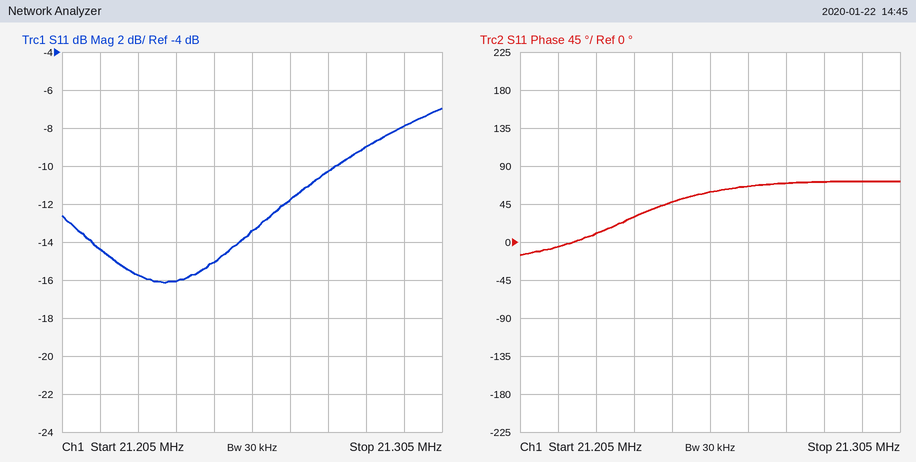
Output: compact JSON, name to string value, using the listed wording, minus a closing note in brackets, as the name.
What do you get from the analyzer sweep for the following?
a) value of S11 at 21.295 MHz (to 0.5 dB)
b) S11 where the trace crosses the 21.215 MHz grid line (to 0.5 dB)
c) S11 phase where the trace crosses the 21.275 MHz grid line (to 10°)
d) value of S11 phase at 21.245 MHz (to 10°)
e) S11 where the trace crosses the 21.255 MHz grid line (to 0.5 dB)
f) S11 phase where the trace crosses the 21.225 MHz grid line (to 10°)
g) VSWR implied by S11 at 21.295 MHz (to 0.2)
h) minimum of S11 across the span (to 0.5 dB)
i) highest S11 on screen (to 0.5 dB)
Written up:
{"value of S11 at 21.295 MHz": "-8.0 dB", "S11 where the trace crosses the 21.215 MHz grid line": "-14.5 dB", "S11 phase where the trace crosses the 21.275 MHz grid line": "70°", "value of S11 phase at 21.245 MHz": "50°", "S11 where the trace crosses the 21.255 MHz grid line": "-13.5 dB", "S11 phase where the trace crosses the 21.225 MHz grid line": "10°", "VSWR implied by S11 at 21.295 MHz": "2.4", "minimum of S11 across the span": "-16.0 dB", "highest S11 on screen": "-7.0 dB"}
